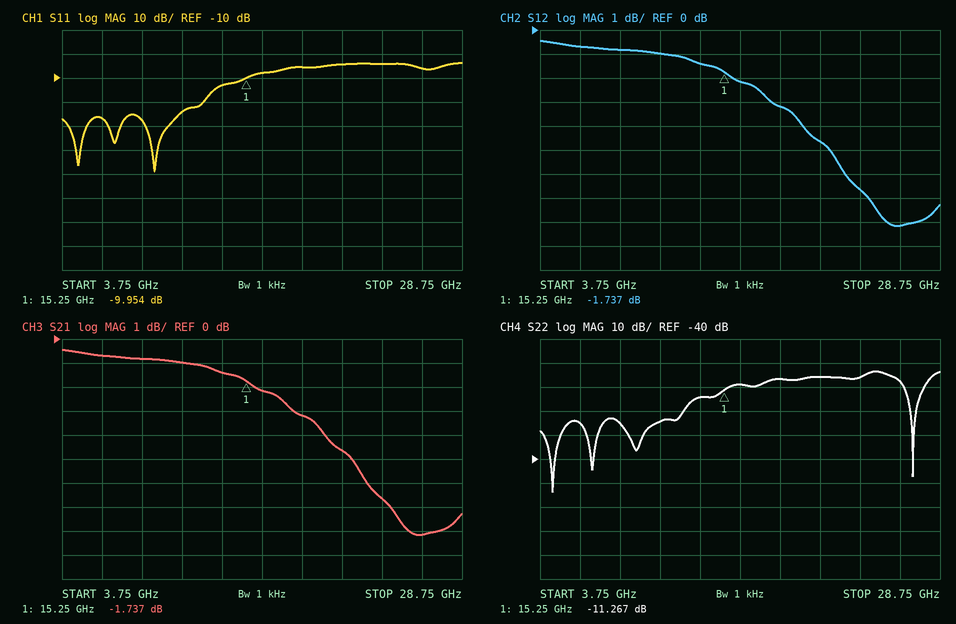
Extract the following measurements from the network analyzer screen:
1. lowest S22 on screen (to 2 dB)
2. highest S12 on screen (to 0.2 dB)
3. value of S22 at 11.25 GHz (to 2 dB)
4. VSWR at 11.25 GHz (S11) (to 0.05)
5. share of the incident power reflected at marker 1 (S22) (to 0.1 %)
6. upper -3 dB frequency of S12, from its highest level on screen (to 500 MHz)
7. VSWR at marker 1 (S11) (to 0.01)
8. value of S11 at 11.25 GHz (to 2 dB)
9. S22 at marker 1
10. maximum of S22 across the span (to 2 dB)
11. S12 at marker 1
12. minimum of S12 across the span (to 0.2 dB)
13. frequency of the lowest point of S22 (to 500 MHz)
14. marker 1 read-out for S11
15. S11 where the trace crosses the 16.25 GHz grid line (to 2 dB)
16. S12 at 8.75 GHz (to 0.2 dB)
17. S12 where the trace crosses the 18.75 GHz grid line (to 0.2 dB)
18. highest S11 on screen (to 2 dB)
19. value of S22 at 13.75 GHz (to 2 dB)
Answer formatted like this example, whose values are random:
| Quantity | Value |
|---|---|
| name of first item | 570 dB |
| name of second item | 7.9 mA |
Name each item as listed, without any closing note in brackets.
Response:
| Quantity | Value |
|---|---|
| lowest S22 on screen | -54 dB |
| highest S12 on screen | -0.4 dB |
| value of S22 at 11.25 GHz | -24 dB |
| VSWR at 11.25 GHz (S11) | 1.15 |
| share of the incident power reflected at marker 1 (S22) | 7.5 % |
| upper -3 dB frequency of S12, from its highest level on screen | 19.5 GHz |
| VSWR at marker 1 (S11) | 1.93 |
| value of S11 at 11.25 GHz | -24 dB |
| S22 at marker 1 | -11.267 dB |
| maximum of S22 across the span | -4 dB |
| S12 at marker 1 | -1.737 dB |
| minimum of S12 across the span | -8.2 dB |
| frequency of the lowest point of S22 | 4.5 GHz |
| marker 1 read-out for S11 | -9.954 dB |
| S11 where the trace crosses the 16.25 GHz grid line | -8 dB |
| S12 at 8.75 GHz | -0.8 dB |
| S12 where the trace crosses the 18.75 GHz grid line | -3.2 dB |
| highest S11 on screen | -4 dB |
| value of S22 at 13.75 GHz | -14 dB |
